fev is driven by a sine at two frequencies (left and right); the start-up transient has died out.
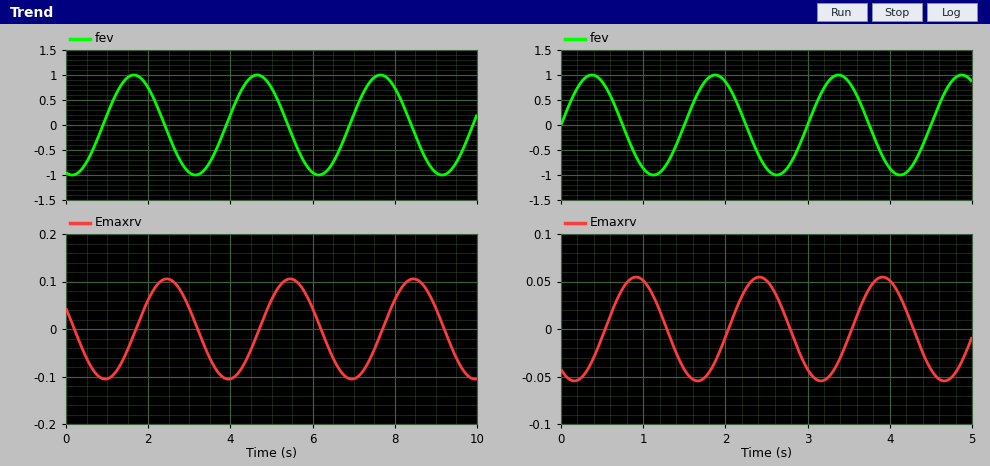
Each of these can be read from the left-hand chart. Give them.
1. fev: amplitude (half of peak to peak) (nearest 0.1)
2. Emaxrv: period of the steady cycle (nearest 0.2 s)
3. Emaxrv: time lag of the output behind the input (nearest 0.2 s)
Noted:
1.0
3.0 s
0.8 s
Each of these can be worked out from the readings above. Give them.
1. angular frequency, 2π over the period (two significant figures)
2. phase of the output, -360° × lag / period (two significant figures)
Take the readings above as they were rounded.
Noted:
2.1 rad/s
-96°
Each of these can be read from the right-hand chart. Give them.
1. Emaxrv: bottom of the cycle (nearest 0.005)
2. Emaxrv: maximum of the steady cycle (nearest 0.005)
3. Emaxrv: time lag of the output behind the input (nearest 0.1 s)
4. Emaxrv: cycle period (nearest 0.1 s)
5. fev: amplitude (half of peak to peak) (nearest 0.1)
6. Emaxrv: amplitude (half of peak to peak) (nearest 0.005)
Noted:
-0.055
0.055
0.5 s
1.5 s
1.0
0.055
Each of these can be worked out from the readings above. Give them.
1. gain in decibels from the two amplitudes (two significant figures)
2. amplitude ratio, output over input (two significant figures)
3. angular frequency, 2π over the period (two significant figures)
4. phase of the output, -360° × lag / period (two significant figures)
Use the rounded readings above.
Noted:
-25 dB
0.055
4.2 rad/s
-120°
